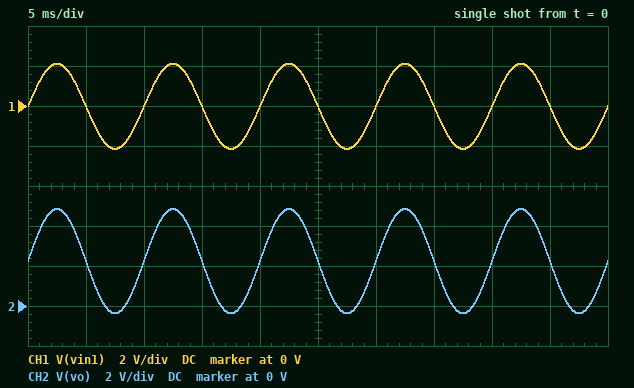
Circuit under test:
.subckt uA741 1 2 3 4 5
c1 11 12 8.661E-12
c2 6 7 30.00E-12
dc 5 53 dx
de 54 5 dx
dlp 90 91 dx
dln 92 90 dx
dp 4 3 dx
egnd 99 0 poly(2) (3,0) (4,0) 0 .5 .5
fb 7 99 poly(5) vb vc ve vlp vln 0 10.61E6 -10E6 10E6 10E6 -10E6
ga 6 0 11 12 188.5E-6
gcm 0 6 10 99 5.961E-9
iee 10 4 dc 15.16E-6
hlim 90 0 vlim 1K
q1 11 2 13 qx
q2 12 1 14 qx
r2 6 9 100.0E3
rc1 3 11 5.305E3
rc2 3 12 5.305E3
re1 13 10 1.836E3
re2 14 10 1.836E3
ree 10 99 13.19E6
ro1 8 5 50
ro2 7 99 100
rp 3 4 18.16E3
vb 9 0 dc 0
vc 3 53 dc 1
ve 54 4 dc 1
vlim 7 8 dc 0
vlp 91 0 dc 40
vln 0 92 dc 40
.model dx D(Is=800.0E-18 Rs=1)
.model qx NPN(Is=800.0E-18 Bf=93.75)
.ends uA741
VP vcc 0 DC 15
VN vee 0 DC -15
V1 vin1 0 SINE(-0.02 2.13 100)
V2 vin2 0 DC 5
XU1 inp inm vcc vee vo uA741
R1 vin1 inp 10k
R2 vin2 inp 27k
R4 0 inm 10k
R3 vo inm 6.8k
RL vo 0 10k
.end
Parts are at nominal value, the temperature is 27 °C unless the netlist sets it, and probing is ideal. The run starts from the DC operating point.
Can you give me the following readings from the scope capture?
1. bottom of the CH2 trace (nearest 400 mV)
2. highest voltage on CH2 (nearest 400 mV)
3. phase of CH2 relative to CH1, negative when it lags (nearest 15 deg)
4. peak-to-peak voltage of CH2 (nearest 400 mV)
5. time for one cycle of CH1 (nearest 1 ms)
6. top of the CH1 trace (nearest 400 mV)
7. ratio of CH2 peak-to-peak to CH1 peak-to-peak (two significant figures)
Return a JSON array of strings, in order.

["-400 mV", "4.8 V", "0 deg", "5.2 V", "10 ms", "2.0 V", "1.2"]
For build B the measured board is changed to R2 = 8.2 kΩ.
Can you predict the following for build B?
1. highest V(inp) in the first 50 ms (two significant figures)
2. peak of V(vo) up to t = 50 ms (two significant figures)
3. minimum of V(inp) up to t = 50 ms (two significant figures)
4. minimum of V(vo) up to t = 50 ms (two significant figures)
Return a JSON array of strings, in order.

["3.7 V", "6.2 V", "1.8 V", "3.0 V"]
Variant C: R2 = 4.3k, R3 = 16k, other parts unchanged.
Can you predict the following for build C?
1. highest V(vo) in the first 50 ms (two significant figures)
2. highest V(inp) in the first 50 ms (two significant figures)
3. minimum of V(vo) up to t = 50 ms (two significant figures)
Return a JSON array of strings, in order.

["11 V", "4.1 V", "7.4 V"]
